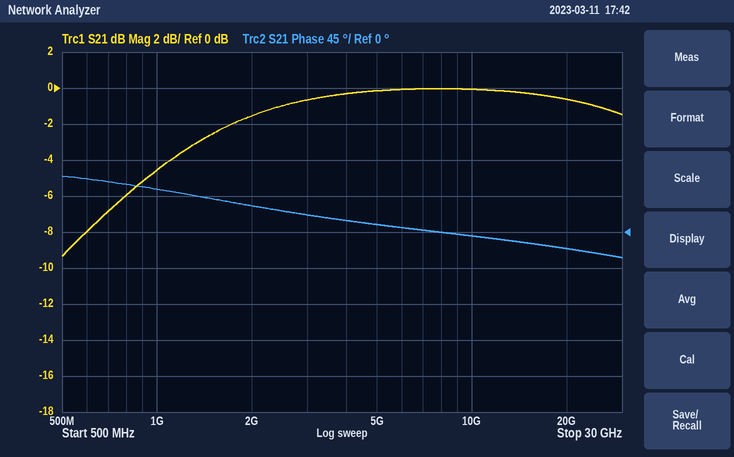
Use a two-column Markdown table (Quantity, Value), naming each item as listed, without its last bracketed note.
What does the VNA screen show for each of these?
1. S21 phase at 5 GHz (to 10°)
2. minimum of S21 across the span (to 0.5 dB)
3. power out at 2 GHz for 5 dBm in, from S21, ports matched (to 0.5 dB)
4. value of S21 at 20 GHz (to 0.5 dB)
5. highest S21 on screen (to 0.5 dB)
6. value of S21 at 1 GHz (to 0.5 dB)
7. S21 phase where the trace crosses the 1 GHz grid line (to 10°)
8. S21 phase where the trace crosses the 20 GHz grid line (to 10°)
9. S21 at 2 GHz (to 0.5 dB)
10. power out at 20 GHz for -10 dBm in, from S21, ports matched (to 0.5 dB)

| Quantity | Value |
|---|---|
| S21 phase at 5 GHz | 10° |
| minimum of S21 across the span | -9.5 dB |
| power out at 2 GHz for 5 dBm in, from S21, ports matched | 3.5 dBm |
| value of S21 at 20 GHz | -0.5 dB |
| highest S21 on screen | 0.0 dB |
| value of S21 at 1 GHz | -4.5 dB |
| S21 phase where the trace crosses the 1 GHz grid line | 50° |
| S21 phase where the trace crosses the 20 GHz grid line | -20° |
| S21 at 2 GHz | -1.5 dB |
| power out at 20 GHz for -10 dBm in, from S21, ports matched | -10.5 dBm |
